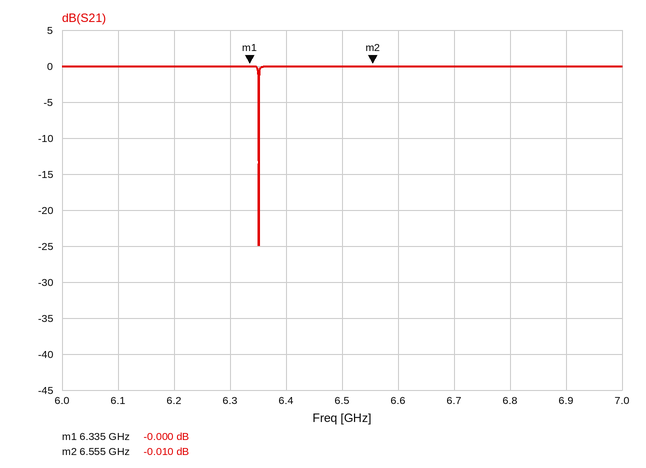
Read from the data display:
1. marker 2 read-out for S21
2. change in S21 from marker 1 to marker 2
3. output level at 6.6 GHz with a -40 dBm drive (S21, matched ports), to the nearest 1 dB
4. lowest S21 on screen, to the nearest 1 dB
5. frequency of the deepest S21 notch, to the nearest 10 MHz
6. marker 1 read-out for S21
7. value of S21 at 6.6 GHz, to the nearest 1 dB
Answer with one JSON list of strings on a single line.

["-0.010 dB", "-0.010 dB", "-40 dBm", "-25 dB", "6.35 GHz", "-0.000 dB", "0 dB"]
